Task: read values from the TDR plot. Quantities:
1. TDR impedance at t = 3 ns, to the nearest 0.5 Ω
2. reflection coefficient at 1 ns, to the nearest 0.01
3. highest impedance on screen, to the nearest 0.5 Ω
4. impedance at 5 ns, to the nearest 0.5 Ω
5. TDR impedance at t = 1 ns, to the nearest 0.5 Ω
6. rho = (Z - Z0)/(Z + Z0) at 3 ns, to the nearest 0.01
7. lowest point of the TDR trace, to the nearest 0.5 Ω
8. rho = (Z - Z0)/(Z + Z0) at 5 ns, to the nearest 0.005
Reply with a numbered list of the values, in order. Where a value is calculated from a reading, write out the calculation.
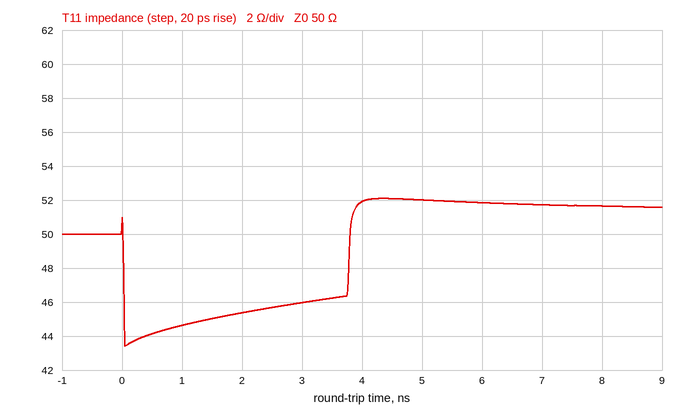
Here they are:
1. 46.0 Ω
2. (44.5 − 50)/(44.5 + 50) ≈ -0.06
3. 52.0 Ω
4. 52.0 Ω
5. 44.5 Ω
6. (46 − 50)/(46 + 50) ≈ -0.04
7. 43.5 Ω
8. (52 − 50)/(52 + 50) ≈ +0.020
